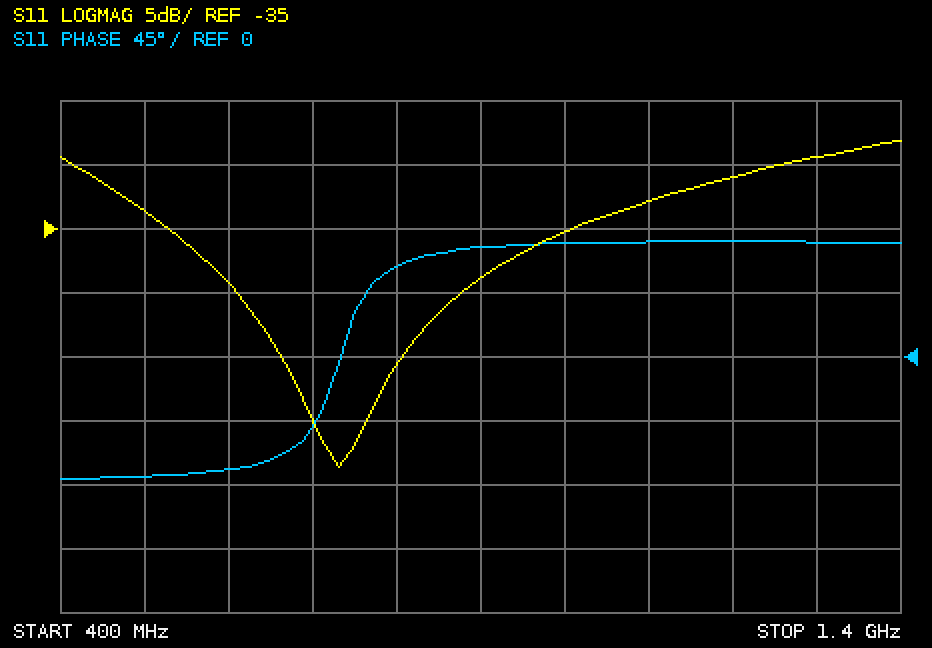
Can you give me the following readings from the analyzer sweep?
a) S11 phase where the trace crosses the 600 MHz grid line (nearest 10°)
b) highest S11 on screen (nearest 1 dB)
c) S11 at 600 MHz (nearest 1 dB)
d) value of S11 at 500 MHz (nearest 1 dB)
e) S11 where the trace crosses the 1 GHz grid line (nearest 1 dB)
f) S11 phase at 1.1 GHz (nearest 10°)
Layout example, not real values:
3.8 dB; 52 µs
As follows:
-80°; -28 dB; -39 dB; -34 dB; -35 dB; 80°
